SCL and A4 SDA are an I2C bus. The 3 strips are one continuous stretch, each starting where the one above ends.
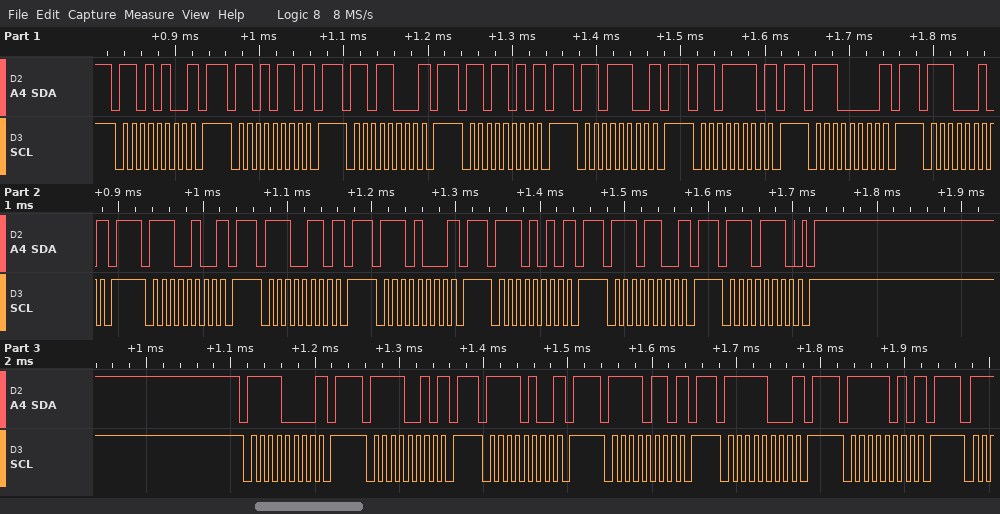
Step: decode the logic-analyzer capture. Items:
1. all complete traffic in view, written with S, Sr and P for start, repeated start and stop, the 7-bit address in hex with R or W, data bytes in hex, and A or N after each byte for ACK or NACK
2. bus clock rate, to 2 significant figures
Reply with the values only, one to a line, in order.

S 6AW N P S 6BW N P S 6CW N P S 6DW N P S 6EW N P S 6FW N P S 70W N P S 71W N P S 72W N P S 73W N P S 74W N P S 75W N P S 76W N P S 77W A P S 78W N P S 79W N P S 7AW N P S 7BW N P S 7CW N P S 7DW N P
100 kHz
